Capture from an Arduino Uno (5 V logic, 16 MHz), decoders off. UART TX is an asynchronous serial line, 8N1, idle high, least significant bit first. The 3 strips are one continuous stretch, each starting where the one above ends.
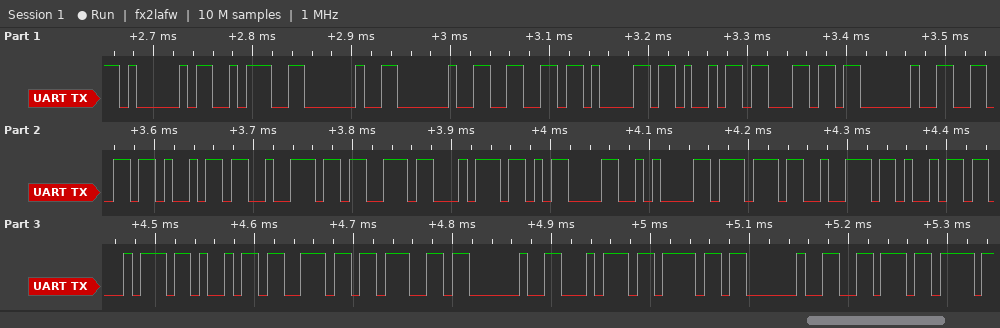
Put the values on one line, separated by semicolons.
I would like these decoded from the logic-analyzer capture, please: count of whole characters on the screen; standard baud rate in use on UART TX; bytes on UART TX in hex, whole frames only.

28; 115200 baud; 0x41 0x3A 0x20 0x20 0x66 0x61 0x69 0x6C 0x20 0x66 0x69 0x72 0x73 0x74 0x0D 0x0A 0x77 0x72 0x69 0x74 0x69 0x6E 0x67 0x20 0x74 0x6F 0x20 0x76
